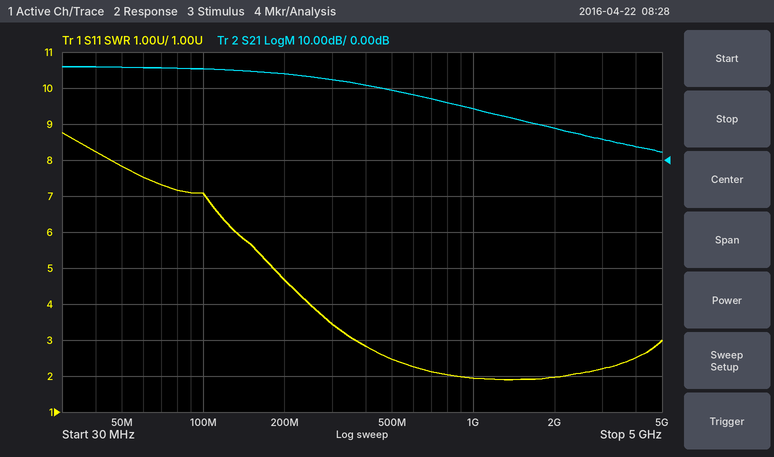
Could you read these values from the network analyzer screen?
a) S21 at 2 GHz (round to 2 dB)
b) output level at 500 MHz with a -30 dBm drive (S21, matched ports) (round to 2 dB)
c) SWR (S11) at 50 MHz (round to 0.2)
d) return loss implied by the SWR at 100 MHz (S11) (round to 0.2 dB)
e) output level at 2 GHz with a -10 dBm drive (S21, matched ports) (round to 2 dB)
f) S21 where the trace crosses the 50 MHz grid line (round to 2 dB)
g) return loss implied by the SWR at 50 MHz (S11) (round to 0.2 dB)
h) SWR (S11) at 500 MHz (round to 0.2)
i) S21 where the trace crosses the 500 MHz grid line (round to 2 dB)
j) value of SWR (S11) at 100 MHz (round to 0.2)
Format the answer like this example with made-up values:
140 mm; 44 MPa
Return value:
8 dB; -10 dBm; 7.8; 2.4 dB; -2 dBm; 26 dB; 2.2 dB; 2.4; 20 dB; 7.0
